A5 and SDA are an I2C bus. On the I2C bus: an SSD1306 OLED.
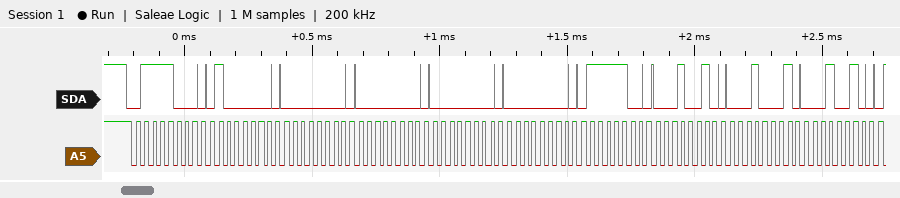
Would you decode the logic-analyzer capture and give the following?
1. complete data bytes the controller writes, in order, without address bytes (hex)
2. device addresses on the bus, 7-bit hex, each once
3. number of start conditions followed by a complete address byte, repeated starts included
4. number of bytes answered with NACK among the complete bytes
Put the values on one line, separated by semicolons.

40 00 00 00 00 7C 12 11 12; 0x3C; 1; 0
